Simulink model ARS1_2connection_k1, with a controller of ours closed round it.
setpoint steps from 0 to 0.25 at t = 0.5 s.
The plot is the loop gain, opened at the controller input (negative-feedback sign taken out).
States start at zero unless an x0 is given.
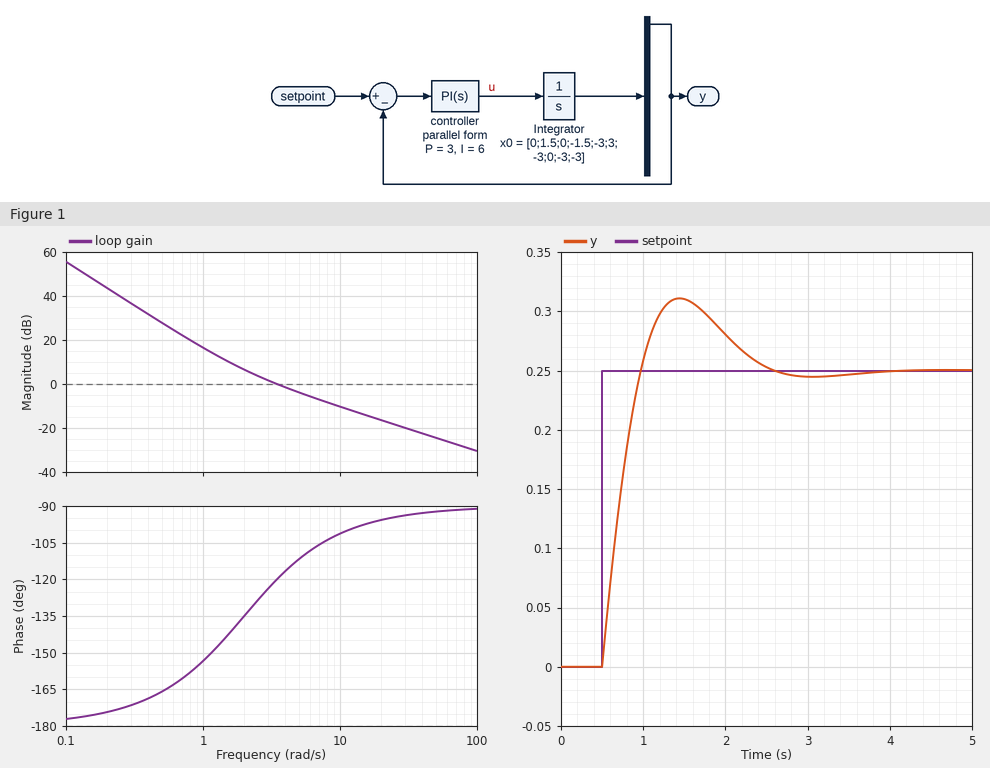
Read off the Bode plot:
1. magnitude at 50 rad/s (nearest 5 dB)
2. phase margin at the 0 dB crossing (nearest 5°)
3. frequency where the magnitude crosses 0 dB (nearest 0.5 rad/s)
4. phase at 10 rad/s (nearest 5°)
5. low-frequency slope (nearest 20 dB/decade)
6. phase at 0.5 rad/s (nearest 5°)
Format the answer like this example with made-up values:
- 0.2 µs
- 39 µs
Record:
- -25 dB
- 60°
- 3.5 rad/s
- -100°
- -40 dB/decade
- -165°
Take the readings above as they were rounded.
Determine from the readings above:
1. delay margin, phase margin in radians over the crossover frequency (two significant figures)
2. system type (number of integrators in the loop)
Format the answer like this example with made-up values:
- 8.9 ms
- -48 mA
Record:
- 0.30 s
- 2
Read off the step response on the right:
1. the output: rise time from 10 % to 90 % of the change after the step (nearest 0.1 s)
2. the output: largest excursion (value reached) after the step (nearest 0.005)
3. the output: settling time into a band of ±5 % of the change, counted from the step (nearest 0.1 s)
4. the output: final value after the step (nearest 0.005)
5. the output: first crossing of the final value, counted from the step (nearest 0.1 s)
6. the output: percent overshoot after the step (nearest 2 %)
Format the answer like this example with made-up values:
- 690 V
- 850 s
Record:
- 0.4 s
- 0.310
- 1.8 s
- 0.250
- 0.5 s
- 24 %
